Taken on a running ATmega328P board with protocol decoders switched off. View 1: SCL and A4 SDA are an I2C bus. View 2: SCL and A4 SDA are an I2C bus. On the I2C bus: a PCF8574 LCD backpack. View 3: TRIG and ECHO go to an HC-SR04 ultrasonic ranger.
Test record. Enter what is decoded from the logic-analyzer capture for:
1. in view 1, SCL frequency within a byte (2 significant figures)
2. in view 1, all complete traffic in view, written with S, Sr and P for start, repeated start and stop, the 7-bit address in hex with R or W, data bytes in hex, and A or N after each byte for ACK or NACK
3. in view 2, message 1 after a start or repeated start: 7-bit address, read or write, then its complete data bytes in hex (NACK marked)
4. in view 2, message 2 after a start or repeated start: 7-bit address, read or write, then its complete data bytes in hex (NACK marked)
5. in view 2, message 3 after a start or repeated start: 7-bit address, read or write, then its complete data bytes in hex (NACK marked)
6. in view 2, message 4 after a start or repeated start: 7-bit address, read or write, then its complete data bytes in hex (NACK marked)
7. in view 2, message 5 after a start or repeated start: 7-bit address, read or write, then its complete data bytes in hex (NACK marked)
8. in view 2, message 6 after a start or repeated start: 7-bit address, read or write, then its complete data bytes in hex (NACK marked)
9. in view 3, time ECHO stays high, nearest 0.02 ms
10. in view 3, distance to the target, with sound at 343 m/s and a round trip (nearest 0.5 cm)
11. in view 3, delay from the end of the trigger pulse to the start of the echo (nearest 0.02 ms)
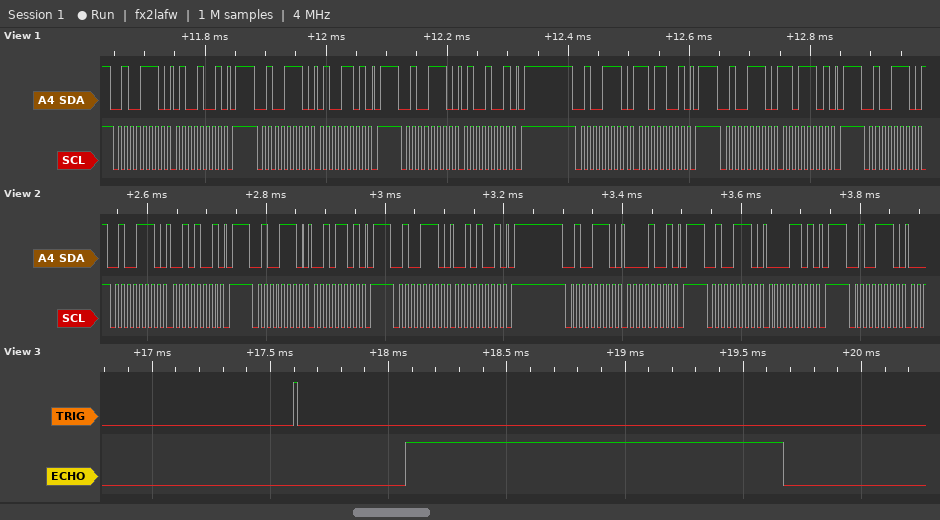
100 kHz
S 27W A 49 A P S 27W A 4D A P S 27W A 49 A P S 27W A D9 A P S 27W A DD A P S 27W A
0x27 write: 29
0x27 write: 2D
0x27 write: 29
0x27 write: 09
0x27 write: 0D
0x27 write
1.60 ms
27.5 cm
0.46 ms
